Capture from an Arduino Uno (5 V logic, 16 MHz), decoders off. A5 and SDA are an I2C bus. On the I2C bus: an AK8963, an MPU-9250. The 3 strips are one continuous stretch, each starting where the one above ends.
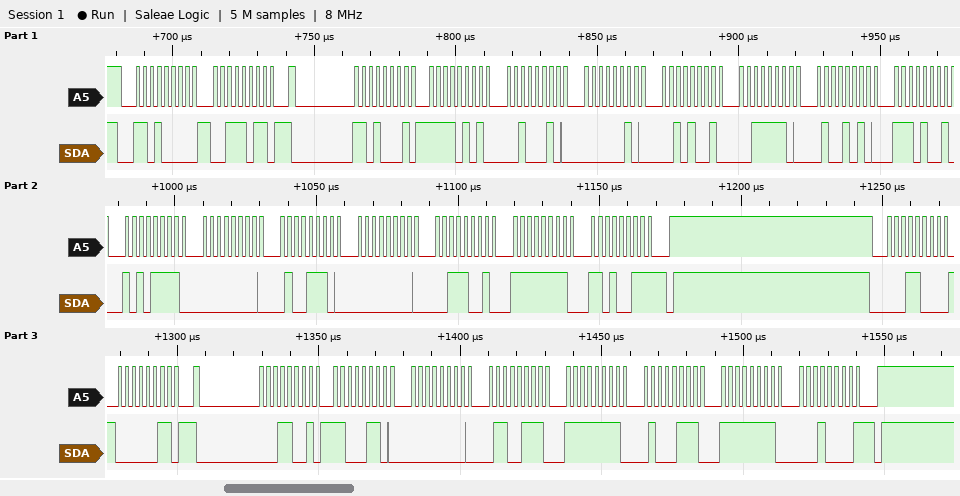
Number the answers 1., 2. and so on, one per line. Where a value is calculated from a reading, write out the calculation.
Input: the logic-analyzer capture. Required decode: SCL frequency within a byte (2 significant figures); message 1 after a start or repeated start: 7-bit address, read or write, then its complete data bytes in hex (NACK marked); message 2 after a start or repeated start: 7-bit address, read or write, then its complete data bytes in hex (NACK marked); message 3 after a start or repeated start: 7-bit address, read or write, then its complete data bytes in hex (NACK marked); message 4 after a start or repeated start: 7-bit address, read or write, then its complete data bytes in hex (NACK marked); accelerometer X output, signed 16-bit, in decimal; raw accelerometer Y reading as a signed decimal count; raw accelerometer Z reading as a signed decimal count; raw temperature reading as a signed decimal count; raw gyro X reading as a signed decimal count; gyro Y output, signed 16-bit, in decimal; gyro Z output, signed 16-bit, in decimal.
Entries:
1. 400 kHz
2. 0x68 write: 3B
3. 0x68 read: F5 22 02 29 3E 4A E9 AF 00 4E 00 39 FF D3 NACK
4. 0x0C write: 03
5. 0x0C read: C6 00 67 FF 47 FF 10 NACK
6. 0xF522 = -2782
7. 0x0229 = 553
8. 0x3E4A = 15946
9. 0xE9AF = -5713
10. 0x004E = 78
11. 0x0039 = 57
12. 0xFFD3 = -45
